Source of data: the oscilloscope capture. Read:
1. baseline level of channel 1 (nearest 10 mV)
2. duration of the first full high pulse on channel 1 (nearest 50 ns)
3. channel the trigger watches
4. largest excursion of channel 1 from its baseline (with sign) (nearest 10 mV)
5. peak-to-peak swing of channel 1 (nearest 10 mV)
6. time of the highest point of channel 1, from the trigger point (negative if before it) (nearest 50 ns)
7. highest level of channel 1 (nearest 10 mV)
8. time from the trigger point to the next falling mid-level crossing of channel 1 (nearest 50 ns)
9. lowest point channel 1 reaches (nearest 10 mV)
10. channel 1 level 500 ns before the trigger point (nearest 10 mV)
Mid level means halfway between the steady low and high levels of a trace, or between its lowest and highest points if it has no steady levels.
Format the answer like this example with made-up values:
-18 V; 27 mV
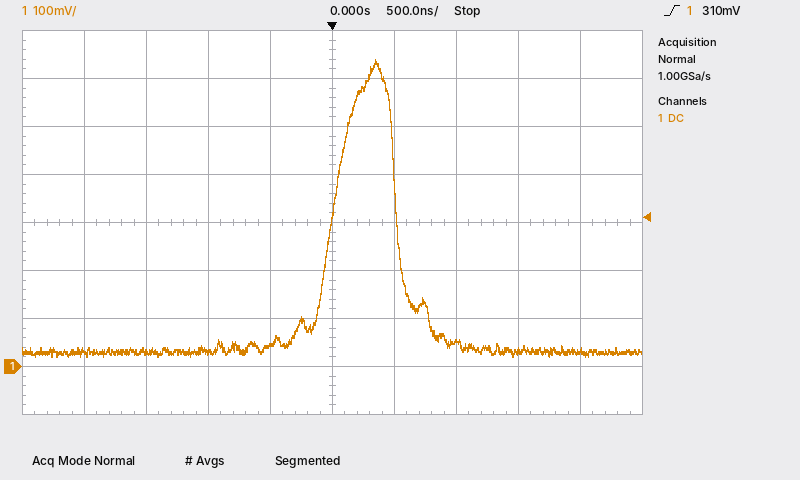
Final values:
30 mV; 500 ns; channel 1; +610 mV; 620 mV; +350 ns; 640 mV; 500 ns; 20 mV; 40 mV
